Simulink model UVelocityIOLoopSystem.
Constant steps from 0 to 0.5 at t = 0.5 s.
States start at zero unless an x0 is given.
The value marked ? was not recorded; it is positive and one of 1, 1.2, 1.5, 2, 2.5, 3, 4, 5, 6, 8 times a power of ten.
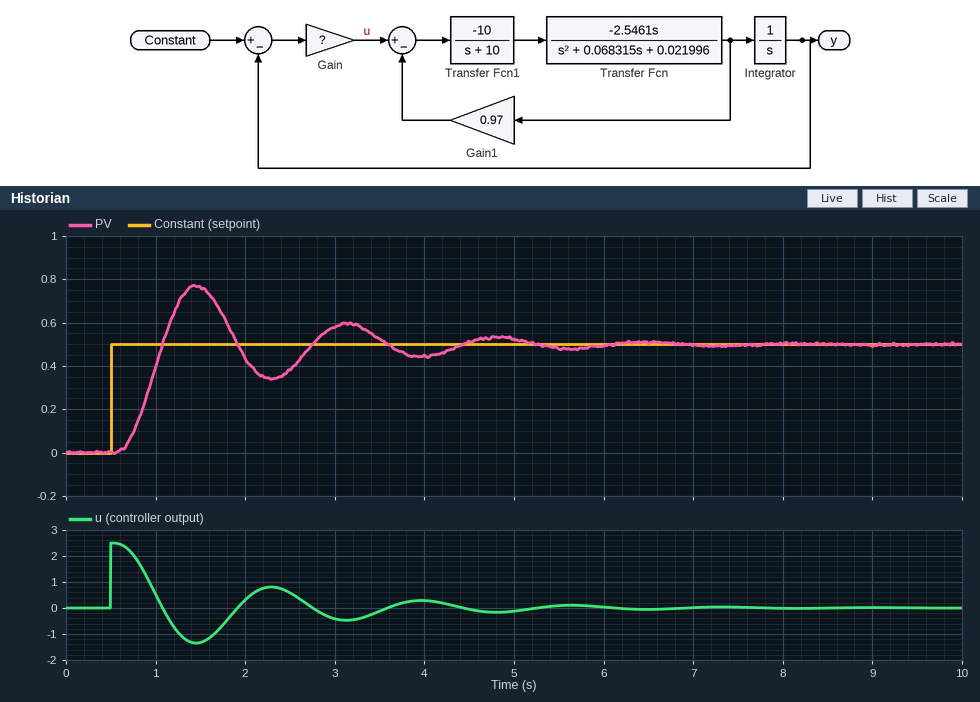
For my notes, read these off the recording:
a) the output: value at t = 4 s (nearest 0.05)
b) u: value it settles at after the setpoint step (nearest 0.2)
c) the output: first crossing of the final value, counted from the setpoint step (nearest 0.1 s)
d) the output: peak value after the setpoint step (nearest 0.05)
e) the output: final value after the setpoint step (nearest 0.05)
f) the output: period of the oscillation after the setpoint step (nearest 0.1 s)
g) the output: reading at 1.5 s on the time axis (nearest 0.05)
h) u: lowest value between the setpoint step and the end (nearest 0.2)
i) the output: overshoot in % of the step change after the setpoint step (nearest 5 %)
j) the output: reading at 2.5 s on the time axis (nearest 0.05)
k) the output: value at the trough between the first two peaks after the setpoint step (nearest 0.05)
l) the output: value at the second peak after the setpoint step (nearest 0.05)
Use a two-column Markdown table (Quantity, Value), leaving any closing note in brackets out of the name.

| Quantity | Value |
|---|---|
| the output: value at t = 4 s | 0.45 |
| u: value it settles at after the setpoint step | 0.0 |
| the output: first crossing of the final value, counted from the setpoint step | 0.6 s |
| the output: peak value after the setpoint step | 0.75 |
| the output: final value after the setpoint step | 0.50 |
| the output: period of the oscillation after the setpoint step | 1.7 s |
| the output: reading at 1.5 s on the time axis | 0.75 |
| u: lowest value between the setpoint step and the end | -1.4 |
| the output: overshoot in % of the step change after the setpoint step | 55 % |
| the output: reading at 2.5 s on the time axis | 0.40 |
| the output: value at the trough between the first two peaks after the setpoint step | 0.35 |
| the output: value at the second peak after the setpoint step | 0.60 |
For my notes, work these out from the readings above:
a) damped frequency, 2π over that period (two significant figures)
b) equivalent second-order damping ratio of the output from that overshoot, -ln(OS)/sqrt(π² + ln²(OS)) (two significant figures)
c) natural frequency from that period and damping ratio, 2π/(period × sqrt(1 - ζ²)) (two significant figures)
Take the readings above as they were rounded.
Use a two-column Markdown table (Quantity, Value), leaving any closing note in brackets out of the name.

| Quantity | Value |
|---|---|
| damped frequency, 2π over that period | 3.7 rad/s |
| equivalent second-order damping ratio of the output from that overshoot, -ln(OS)/sqrt(π² + ln²(OS)) | 0.19 |
| natural frequency from that period and damping ratio, 2π/(period × sqrt(1 - ζ²)) | 3.8 rad/s |
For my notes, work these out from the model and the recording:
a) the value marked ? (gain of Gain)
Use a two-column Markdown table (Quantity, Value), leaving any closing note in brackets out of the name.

| Quantity | Value |
|---|---|
| the value marked ? | 5 |
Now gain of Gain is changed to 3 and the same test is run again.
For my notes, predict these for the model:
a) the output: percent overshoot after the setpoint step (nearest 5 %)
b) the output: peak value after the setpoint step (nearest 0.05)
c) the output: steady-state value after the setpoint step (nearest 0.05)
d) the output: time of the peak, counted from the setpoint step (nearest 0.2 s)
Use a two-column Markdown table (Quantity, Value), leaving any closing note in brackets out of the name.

| Quantity | Value |
|---|---|
| the output: percent overshoot after the setpoint step | 30 % |
| the output: peak value after the setpoint step | 0.65 |
| the output: steady-state value after the setpoint step | 0.50 |
| the output: time of the peak, counted from the setpoint step | 1.2 s |
